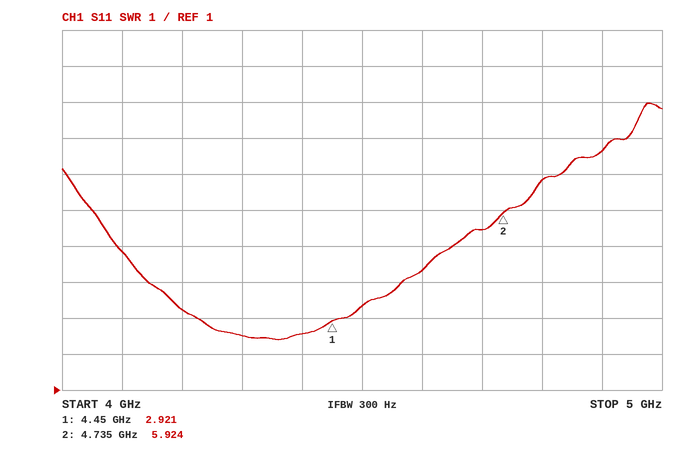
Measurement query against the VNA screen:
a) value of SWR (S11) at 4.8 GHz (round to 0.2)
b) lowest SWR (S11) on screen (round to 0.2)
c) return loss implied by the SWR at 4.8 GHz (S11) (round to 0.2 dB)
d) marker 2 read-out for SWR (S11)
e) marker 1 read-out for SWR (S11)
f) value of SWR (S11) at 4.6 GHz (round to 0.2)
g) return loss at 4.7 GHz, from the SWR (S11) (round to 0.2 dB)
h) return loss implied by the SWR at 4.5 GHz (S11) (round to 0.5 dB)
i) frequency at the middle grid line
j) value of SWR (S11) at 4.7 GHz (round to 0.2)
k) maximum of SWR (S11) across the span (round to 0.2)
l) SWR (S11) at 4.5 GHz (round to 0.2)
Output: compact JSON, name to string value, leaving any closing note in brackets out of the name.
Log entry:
{"value of SWR (S11) at 4.8 GHz": "6.8", "lowest SWR (S11) on screen": "2.4", "return loss implied by the SWR at 4.8 GHz (S11)": "2.6 dB", "marker 2 read-out for SWR": "5.924", "marker 1 read-out for SWR": "2.921", "value of SWR (S11) at 4.6 GHz": "4.4", "return loss at 4.7 GHz, from the SWR (S11)": "3.2 dB", "return loss implied by the SWR at 4.5 GHz (S11)": "5.5 dB", "frequency at the middle grid line": "4.5 GHz", "value of SWR (S11) at 4.7 GHz": "5.4", "maximum of SWR (S11) across the span": "9.0", "SWR (S11) at 4.5 GHz": "3.4"}
